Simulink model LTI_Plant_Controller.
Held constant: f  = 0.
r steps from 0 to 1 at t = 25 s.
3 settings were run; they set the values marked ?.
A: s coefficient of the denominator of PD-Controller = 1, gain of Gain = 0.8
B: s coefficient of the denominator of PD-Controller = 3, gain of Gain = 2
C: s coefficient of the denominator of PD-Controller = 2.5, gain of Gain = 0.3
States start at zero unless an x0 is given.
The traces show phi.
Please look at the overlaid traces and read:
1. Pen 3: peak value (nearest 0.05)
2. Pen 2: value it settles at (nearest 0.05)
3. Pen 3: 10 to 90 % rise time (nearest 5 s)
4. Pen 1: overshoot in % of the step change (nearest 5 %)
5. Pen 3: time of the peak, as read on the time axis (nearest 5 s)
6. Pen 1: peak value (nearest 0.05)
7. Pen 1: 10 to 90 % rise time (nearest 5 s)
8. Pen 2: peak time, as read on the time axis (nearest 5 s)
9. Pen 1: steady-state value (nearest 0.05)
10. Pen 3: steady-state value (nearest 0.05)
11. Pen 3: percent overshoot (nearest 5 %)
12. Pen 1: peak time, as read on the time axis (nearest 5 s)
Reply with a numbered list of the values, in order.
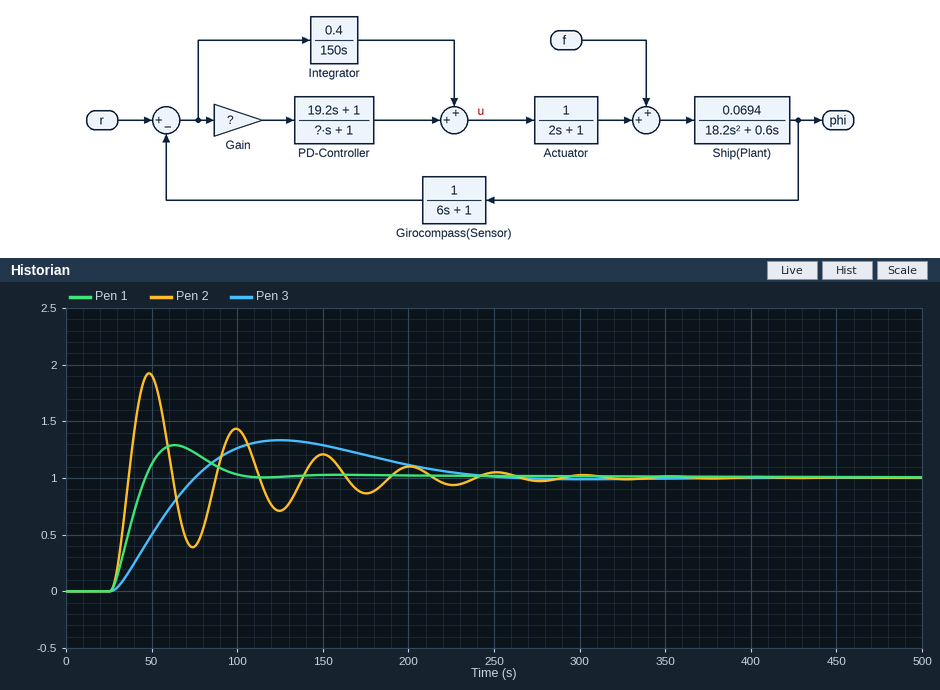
1. 1.35
2. 1.00
3. 35 s
4. 30 %
5. 125 s
6. 1.30
7. 15 s
8. 50 s
9. 1.00
10. 1.00
11. 35 %
12. 65 s
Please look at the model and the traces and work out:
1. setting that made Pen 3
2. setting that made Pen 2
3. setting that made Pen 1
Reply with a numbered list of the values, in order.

1. C
2. B
3. A
